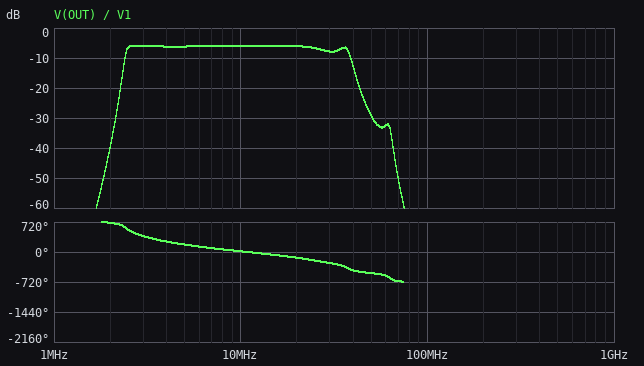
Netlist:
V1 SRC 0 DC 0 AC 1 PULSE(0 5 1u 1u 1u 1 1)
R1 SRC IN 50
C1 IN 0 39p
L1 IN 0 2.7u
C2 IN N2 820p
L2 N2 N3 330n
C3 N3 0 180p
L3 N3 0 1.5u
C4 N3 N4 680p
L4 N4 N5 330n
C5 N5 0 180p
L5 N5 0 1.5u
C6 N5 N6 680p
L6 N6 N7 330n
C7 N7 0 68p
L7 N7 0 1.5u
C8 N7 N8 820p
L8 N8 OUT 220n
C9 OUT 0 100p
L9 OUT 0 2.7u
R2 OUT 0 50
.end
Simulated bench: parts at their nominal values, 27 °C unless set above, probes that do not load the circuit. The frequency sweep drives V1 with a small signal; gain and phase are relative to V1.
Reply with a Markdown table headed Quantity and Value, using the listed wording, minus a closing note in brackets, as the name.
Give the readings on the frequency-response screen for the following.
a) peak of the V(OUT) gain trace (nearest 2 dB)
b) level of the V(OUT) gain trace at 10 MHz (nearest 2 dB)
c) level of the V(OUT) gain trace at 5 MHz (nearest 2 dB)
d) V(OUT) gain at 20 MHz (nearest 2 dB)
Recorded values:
| Quantity | Value |
|---|---|
| peak of the V(OUT) gain trace | -6 dB |
| level of the V(OUT) gain trace at 10 MHz | -6 dB |
| level of the V(OUT) gain trace at 5 MHz | -6 dB |
| V(OUT) gain at 20 MHz | -6 dB |
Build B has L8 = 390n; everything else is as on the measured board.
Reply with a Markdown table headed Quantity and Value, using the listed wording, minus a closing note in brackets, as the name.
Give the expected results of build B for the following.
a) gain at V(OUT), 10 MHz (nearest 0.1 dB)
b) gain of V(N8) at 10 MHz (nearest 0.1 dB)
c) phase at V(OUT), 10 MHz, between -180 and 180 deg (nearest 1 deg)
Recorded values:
| Quantity | Value |
|---|---|
| gain at V(OUT), 10 MHz | -6.2 dB |
| gain of V(N8) at 10 MHz | -5.3 dB |
| phase at V(OUT), 10 MHz, between -180 and 180 deg | 11 deg |
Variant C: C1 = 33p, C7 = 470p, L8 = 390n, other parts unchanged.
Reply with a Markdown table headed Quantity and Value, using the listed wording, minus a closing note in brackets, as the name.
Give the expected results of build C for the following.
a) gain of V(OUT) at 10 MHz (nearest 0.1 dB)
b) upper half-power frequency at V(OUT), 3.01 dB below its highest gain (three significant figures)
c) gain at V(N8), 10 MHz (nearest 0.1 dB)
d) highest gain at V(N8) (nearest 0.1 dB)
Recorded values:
| Quantity | Value |
|---|---|
| gain of V(OUT) at 10 MHz | -6.7 dB |
| upper half-power frequency at V(OUT), 3.01 dB below its highest gain | 25.3 MHz |
| gain at V(N8), 10 MHz | -5.8 dB |
| highest gain at V(N8) | -4.9 dB |
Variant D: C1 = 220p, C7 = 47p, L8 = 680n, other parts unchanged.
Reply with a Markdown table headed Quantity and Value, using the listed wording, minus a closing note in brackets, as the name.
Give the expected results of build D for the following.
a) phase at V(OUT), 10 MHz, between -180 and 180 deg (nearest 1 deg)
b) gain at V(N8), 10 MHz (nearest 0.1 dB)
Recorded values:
| Quantity | Value |
|---|---|
| phase at V(OUT), 10 MHz, between -180 and 180 deg | -13 deg |
| gain at V(N8), 10 MHz | -3.8 dB |
